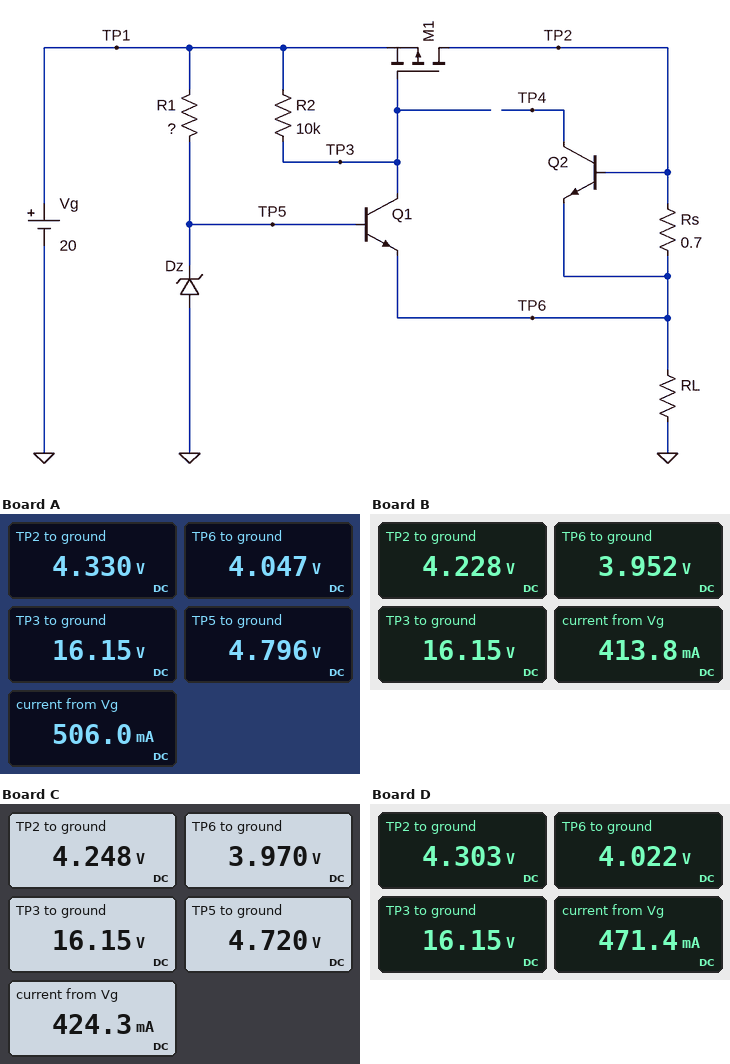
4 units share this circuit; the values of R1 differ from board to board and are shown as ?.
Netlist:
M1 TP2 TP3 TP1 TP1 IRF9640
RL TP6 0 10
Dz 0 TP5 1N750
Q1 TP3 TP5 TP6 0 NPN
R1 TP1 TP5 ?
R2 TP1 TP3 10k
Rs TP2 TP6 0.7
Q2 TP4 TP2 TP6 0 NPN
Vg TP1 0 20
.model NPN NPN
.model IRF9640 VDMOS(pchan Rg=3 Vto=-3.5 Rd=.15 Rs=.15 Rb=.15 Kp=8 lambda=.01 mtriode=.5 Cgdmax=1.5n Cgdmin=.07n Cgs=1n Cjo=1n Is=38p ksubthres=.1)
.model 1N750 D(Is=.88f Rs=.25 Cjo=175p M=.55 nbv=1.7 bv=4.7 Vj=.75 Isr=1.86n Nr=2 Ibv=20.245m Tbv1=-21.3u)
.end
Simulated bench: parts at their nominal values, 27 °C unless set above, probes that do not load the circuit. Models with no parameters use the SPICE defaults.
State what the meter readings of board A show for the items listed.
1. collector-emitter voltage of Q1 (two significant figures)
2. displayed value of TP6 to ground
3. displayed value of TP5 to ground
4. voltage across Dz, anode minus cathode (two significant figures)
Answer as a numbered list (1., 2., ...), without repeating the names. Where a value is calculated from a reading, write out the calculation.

1. 16.15 V - 4.047 V = 12 V
2. 4.047 V
3. 4.796 V
4. 0 V - 4.796 V = -4.8 V
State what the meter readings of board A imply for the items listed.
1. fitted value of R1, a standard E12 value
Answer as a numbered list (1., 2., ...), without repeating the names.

1. 150 Ω
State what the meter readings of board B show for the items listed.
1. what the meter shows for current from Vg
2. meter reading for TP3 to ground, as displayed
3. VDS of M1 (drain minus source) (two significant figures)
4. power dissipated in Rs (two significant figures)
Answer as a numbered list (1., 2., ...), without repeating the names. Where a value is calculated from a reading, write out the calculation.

1. 413.8 mA
2. 16.15 V
3. 4.228 V - 20 V = -16 V
4. (4.228 V - 3.952 V)^2 / 700 mΩ = 110 mW
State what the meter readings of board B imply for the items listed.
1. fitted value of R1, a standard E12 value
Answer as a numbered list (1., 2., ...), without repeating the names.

1. 820 Ω
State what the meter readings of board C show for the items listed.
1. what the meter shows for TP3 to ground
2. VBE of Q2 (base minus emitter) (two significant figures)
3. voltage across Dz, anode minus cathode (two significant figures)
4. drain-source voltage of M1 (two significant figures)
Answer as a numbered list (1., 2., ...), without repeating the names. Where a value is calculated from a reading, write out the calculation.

1. 16.15 V
2. 4.248 V - 3.97 V = 280 mV
3. 0 V - 4.72 V = -4.7 V
4. 4.248 V - 20 V = -16 V
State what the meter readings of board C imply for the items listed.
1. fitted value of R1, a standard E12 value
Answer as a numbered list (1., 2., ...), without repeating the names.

1. 560 Ω
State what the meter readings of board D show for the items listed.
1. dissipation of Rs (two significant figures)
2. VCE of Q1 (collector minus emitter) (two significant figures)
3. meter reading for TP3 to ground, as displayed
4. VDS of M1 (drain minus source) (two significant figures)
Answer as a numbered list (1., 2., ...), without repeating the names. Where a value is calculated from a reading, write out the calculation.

1. (4.303 V - 4.022 V)^2 / 700 mΩ = 110 mW
2. 16.15 V - 4.022 V = 12 V
3. 16.15 V
4. 4.303 V - 20 V = -16 V
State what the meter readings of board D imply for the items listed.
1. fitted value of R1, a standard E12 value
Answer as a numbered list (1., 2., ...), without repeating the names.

1. 220 Ω
